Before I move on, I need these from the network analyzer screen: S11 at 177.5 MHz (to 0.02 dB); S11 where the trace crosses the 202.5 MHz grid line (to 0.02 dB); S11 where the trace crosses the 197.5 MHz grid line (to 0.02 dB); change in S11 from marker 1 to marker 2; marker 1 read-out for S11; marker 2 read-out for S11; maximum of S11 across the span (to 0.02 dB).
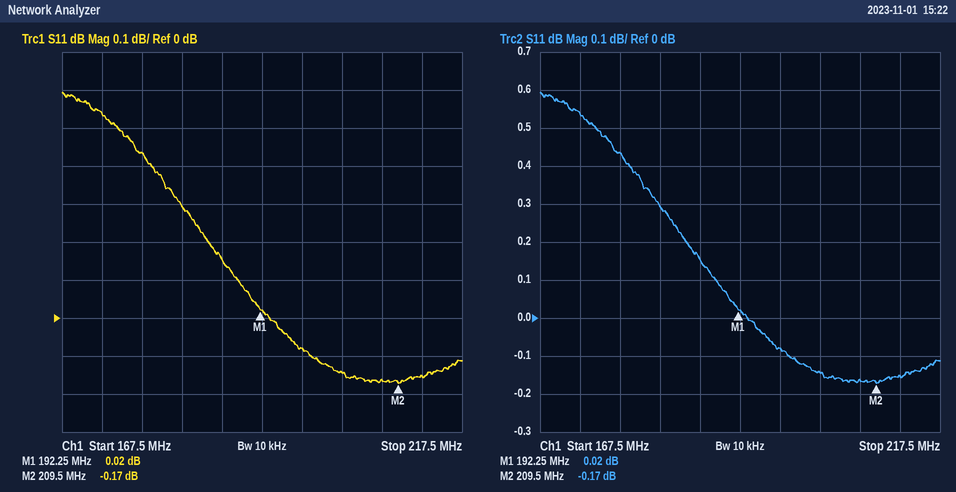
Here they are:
0.44 dB
-0.14 dB
-0.08 dB
-0.19 dB
0.02 dB
-0.17 dB
0.60 dB
